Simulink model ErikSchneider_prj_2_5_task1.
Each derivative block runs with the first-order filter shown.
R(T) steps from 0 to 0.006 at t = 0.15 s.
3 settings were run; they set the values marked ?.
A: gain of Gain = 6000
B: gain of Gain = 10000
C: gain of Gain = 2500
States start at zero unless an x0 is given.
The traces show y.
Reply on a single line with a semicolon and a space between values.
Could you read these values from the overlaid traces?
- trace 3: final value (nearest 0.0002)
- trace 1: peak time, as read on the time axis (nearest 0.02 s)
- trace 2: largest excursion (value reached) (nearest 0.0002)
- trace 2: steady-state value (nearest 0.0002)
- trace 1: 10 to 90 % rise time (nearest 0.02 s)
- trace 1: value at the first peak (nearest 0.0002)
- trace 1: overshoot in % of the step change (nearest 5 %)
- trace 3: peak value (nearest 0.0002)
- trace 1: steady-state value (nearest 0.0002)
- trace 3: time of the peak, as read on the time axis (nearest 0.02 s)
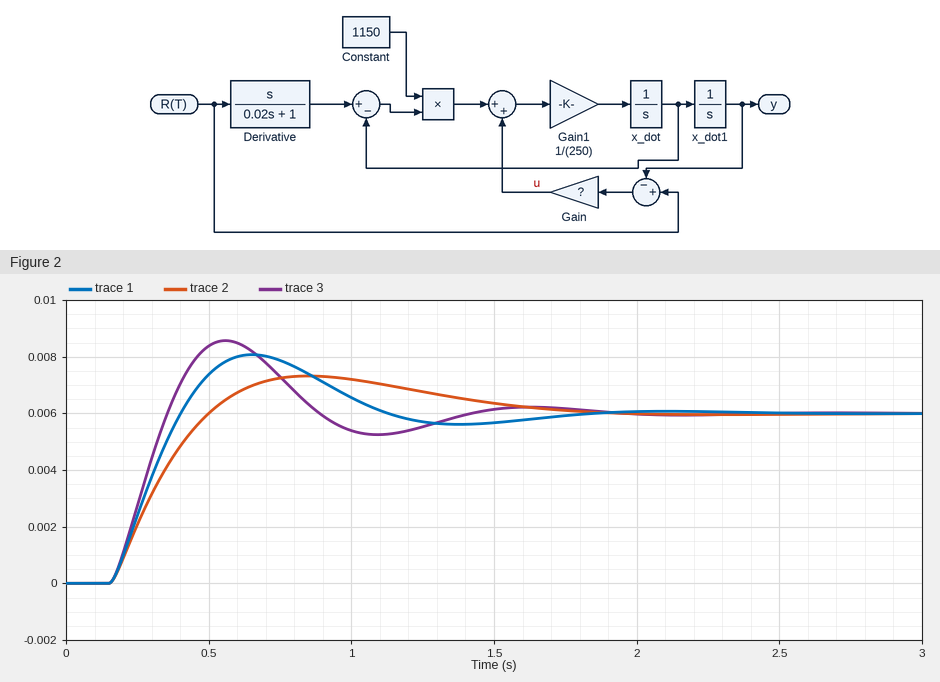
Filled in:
0.0060; 0.66 s; 0.0074; 0.0060; 0.18 s; 0.0080; 35 %; 0.0086; 0.0060; 0.56 s
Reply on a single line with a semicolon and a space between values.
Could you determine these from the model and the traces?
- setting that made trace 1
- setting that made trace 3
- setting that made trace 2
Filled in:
A; B; C
